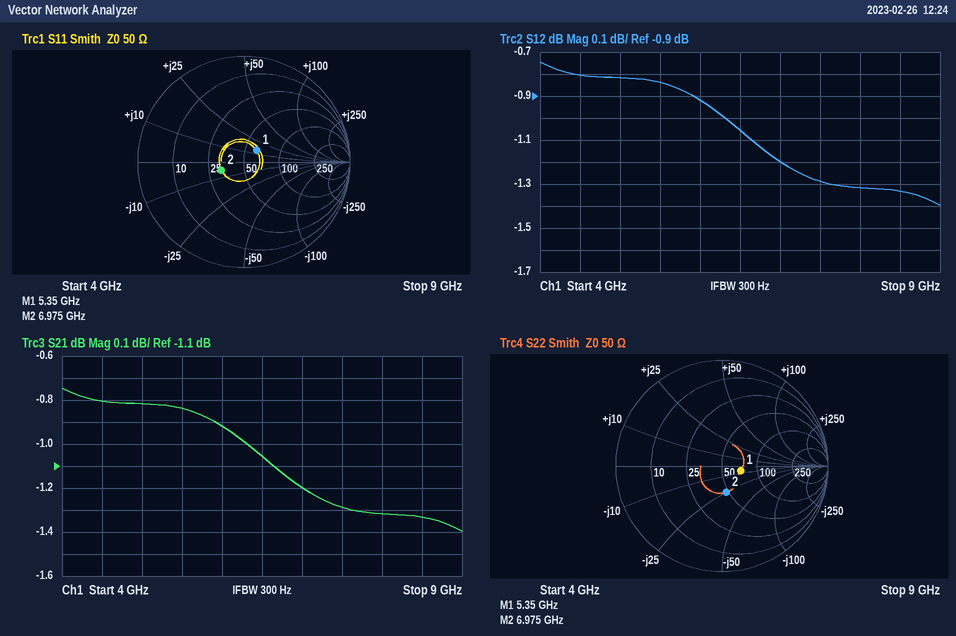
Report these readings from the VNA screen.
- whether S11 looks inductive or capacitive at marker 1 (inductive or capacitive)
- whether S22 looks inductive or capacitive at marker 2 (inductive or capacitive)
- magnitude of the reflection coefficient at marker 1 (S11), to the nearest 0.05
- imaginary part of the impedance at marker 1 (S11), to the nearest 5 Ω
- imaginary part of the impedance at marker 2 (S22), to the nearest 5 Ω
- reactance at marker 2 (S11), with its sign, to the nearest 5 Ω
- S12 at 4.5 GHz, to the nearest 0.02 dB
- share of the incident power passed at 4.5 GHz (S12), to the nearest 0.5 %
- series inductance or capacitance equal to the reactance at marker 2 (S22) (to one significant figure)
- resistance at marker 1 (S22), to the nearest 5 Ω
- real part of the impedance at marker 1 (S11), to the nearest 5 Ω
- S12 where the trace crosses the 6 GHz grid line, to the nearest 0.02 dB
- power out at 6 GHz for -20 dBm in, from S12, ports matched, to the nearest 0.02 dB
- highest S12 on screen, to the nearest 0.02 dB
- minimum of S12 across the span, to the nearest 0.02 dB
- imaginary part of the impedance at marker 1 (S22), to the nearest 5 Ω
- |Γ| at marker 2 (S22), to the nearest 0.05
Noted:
inductive
capacitive
0.15
+15 Ω
-25 Ω
-5 Ω
-0.80 dB
83.0 %
900 fF
70 Ω
60 Ω
-0.92 dB
-20.92 dBm
-0.74 dB
-1.40 dB
-5 Ω
0.25
